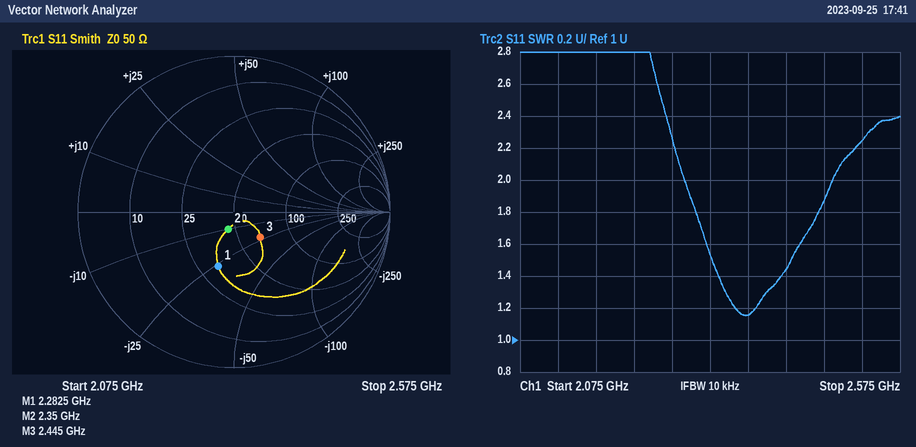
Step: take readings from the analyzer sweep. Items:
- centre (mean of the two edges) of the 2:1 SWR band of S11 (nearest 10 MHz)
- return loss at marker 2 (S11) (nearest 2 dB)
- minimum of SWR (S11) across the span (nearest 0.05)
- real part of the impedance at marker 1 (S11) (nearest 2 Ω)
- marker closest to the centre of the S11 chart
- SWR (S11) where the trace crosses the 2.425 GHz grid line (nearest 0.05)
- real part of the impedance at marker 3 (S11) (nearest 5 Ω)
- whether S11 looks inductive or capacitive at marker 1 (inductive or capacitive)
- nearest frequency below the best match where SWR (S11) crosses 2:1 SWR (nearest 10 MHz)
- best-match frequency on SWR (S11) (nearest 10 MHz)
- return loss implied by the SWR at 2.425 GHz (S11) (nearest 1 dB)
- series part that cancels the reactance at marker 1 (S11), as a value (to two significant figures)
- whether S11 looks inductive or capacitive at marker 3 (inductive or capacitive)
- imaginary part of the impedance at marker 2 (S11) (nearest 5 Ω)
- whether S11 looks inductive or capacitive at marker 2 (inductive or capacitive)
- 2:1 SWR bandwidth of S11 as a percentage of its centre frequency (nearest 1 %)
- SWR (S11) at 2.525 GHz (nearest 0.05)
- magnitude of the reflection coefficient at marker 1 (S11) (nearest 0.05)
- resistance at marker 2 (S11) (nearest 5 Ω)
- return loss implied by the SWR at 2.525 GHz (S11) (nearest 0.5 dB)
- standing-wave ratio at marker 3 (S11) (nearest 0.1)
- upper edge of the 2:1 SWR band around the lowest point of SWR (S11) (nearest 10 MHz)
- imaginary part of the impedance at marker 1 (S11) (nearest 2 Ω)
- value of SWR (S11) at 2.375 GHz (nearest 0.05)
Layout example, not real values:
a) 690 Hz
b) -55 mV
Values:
a) 2.39 GHz
b) 18 dB
c) 1.15
d) 32 Ω
e) marker 2
f) 1.45
g) 65 Ω
h) capacitive
i) 2.29 GHz
j) 2.37 GHz
k) 15 dB
l) 1.8 nH
m) capacitive
n) -10 Ω
o) capacitive
p) 8 %
q) 2.25
r) 0.35
s) 45 Ω
t) 8.5 dB
u) 1.6
v) 2.49 GHz
w) -26 Ω
x) 1.15
